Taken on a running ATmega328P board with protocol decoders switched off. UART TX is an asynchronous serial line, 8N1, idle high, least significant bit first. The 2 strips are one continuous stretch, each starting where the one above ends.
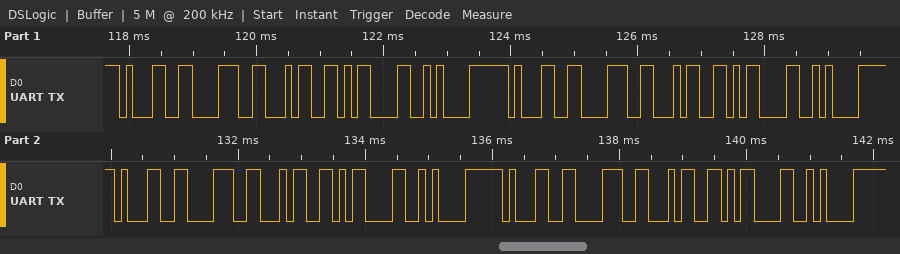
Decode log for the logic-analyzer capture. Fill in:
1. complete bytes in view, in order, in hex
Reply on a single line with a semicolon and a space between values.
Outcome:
0x31 0x38 0x34 0x0D 0x0A 0x31 0x38 0x34 0x0D 0x0A 0x31 0x38 0x34 0x0D 0x0A 0x31 0x38 0x34 0x0D 0x0A
